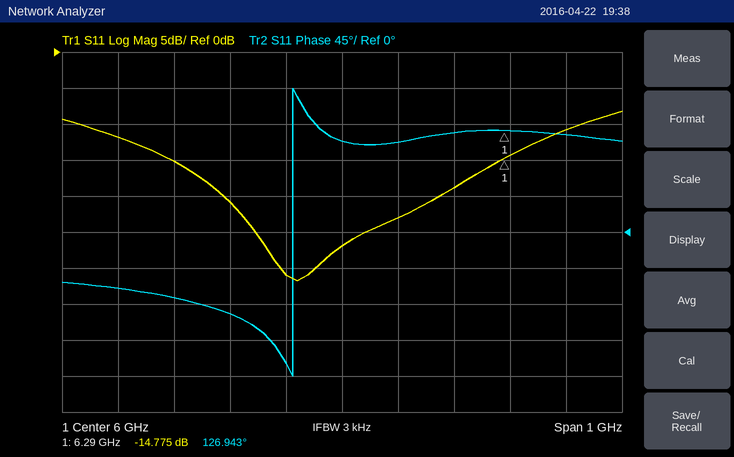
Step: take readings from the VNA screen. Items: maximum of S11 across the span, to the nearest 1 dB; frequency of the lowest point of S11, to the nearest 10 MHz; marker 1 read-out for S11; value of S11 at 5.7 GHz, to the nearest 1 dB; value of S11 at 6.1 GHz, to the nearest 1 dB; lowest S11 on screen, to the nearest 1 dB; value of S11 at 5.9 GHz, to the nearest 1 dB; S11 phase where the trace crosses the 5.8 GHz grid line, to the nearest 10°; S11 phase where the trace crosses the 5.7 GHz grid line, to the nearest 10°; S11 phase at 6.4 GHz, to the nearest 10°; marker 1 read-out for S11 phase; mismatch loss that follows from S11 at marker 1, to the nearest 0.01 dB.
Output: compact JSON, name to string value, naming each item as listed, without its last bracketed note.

{"maximum of S11 across the span, to the nearest 1 dB": "-8 dB", "frequency of the lowest point of S11, to the nearest 10 MHz": "5.92 GHz", "marker 1 read-out for S11": "-14.775 dB", "value of S11 at 5.7 GHz, to the nearest 1 dB": "-15 dB", "value of S11 at 6.1 GHz, to the nearest 1 dB": "-23 dB", "lowest S11 on screen, to the nearest 1 dB": "-32 dB", "value of S11 at 5.9 GHz, to the nearest 1 dB": "-31 dB", "S11 phase where the trace crosses the 5.8 GHz grid line, to the nearest 10°": "-100°", "S11 phase where the trace crosses the 5.7 GHz grid line, to the nearest 10°": "-80°", "S11 phase at 6.4 GHz, to the nearest 10°": "120°", "marker 1 read-out for S11 phase": "126.943°", "mismatch loss that follows from S11 at marker 1, to the nearest 0.01 dB": "0.15 dB"}
